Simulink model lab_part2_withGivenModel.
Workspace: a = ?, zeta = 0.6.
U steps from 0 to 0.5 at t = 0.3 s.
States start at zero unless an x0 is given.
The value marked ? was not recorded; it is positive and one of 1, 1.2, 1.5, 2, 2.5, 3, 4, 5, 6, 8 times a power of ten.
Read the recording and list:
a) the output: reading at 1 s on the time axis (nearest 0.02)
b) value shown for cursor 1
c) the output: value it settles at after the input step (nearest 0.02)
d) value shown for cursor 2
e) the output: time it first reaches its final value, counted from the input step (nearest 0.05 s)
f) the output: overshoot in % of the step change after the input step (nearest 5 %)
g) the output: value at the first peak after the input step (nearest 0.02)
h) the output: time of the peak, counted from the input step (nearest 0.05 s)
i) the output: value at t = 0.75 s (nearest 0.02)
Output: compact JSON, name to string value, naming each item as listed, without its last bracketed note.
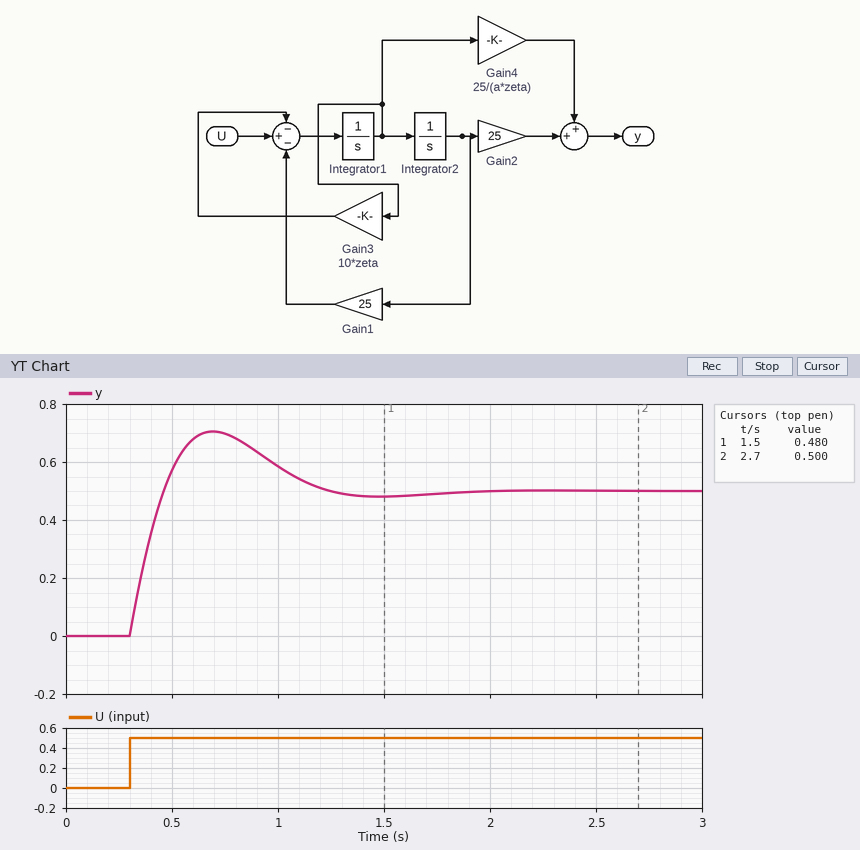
{"the output: reading at 1 s on the time axis": "0.58", "value shown for cursor 1": "0.480", "the output: value it settles at after the input step": "0.50", "value shown for cursor 2": "0.500", "the output: time it first reaches its final value, counted from the input step": "0.15 s", "the output: overshoot in % of the step change after the input step": "40 %", "the output: value at the first peak after the input step": "0.70", "the output: time of the peak, counted from the input step": "0.40 s", "the output: value at t = 0.75 s": "0.70"}
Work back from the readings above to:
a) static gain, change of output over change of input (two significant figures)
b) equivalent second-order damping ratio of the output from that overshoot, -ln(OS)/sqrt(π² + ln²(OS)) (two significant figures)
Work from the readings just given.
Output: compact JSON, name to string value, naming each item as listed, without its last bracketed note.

{"static gain, change of output over change of input": "1.0", "equivalent second-order damping ratio of the output from that overshoot, -ln(OS)/sqrt(π² + ln²(OS))": "0.28"}
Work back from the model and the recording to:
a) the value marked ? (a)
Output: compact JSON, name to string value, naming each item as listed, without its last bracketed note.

{"the value marked ?": "5"}
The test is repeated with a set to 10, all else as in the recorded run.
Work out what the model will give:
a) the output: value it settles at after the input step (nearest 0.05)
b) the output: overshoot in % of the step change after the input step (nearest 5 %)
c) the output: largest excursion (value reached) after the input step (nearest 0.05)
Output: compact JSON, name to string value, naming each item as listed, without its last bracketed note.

{"the output: value it settles at after the input step": "0.50", "the output: overshoot in % of the step change after the input step": "15 %", "the output: largest excursion (value reached) after the input step": "0.60"}
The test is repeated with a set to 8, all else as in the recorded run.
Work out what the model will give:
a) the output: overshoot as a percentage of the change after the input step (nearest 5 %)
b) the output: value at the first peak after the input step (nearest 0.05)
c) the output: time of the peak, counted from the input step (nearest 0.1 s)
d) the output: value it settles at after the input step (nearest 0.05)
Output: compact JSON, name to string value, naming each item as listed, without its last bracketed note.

{"the output: overshoot as a percentage of the change after the input step": "20 %", "the output: value at the first peak after the input step": "0.60", "the output: time of the peak, counted from the input step": "0.5 s", "the output: value it settles at after the input step": "0.50"}
